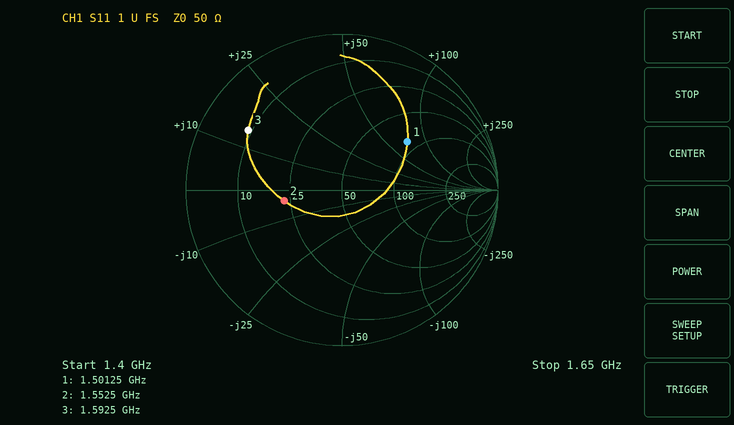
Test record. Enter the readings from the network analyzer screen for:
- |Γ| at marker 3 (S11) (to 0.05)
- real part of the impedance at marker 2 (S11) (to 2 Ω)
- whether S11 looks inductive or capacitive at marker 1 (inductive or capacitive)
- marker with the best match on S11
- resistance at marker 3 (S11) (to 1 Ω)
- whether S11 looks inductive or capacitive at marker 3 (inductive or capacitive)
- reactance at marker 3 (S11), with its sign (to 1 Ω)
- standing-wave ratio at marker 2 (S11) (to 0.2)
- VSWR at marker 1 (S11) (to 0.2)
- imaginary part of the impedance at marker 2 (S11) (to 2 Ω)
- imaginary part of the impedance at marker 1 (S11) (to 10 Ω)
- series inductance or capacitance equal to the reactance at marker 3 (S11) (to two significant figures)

0.70
22 Ω
inductive
marker 2
9 Ω
inductive
+14 Ω
2.2
3.2
-4 Ω
+70 Ω
1.4 nH
